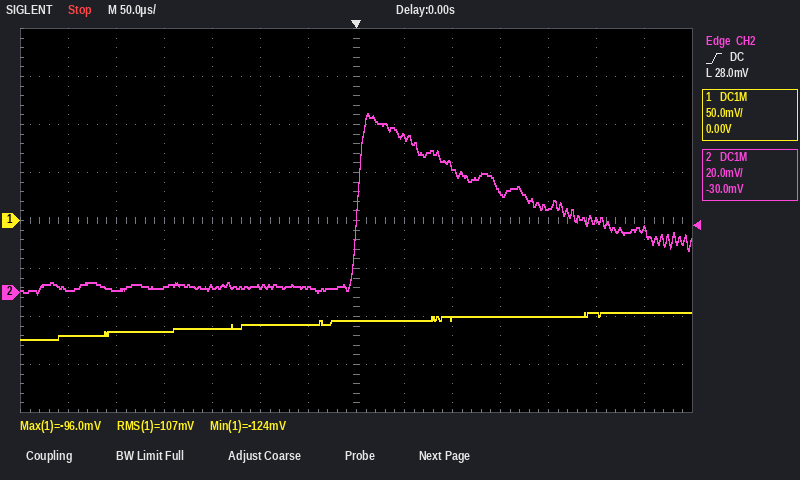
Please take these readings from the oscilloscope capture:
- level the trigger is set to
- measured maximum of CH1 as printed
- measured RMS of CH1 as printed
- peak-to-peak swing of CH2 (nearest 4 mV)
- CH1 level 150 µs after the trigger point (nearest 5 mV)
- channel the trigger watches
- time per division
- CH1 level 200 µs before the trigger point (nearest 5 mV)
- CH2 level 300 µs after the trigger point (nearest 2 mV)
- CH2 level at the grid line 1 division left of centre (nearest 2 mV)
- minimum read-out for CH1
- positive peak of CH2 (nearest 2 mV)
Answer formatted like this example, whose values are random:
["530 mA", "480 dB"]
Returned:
["28.0 mV", "-96.0 mV", "107 mV", "76 mV", "-100 mV", "CH2", "50 µs", "-115 mV", "26 mV", "2 mV", "-124 mV", "74 mV"]
